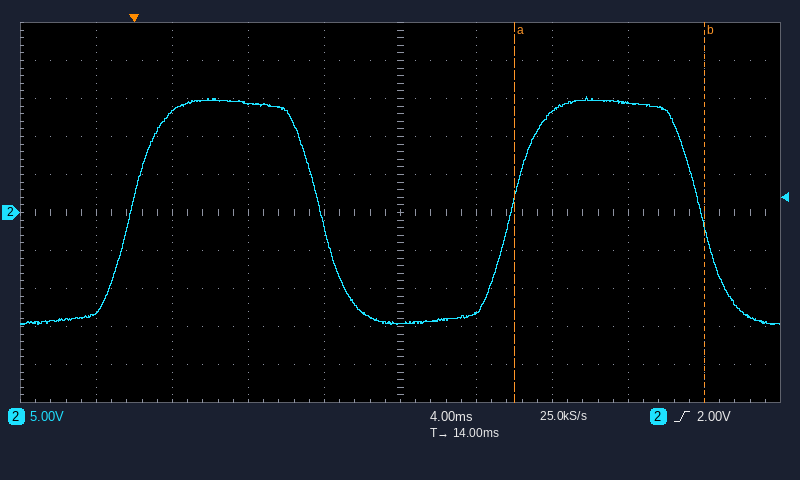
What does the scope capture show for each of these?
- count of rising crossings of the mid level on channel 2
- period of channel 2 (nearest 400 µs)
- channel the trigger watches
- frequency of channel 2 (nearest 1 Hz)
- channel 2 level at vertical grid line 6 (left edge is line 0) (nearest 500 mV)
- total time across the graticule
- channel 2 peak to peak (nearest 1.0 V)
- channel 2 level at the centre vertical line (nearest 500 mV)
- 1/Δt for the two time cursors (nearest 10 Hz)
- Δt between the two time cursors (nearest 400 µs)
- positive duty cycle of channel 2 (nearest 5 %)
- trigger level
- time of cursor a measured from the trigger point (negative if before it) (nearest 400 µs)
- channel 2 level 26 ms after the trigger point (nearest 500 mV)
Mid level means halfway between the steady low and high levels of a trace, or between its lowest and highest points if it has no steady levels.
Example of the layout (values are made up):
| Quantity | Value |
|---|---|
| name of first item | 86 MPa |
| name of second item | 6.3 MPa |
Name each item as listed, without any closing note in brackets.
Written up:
| Quantity | Value |
|---|---|
| count of rising crossings of the mid level on channel 2 | 2 |
| period of channel 2 | 20.0 ms |
| channel the trigger watches | channel 2 |
| frequency of channel 2 | 50 Hz |
| channel 2 level at vertical grid line 6 (left edge is line 0) | -13.0 V |
| total time across the graticule | 40 ms |
| channel 2 peak to peak | 30.0 V |
| channel 2 level at the centre vertical line | -14.5 V |
| 1/Δt for the two time cursors | 100 Hz |
| Δt between the two time cursors | 10.0 ms |
| positive duty cycle of channel 2 | 50 % |
| trigger level | 2.00 V |
| time of cursor a measured from the trigger point (negative if before it) | +20.0 ms |
| channel 2 level 26 ms after the trigger point | 14.5 V |
